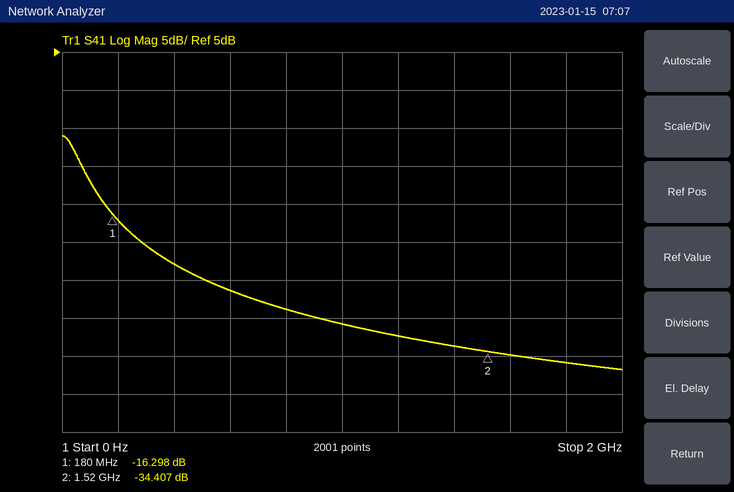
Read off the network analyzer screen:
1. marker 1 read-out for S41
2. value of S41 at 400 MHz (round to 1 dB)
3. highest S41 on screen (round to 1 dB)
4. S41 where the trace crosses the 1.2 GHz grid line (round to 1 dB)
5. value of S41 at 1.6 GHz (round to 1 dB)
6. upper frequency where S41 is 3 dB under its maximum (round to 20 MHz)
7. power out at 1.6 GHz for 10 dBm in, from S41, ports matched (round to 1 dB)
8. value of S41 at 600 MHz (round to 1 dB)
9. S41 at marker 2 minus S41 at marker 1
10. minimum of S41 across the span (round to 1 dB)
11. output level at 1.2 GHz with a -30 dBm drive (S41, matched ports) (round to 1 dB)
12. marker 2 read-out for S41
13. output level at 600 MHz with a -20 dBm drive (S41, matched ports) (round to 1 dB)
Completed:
-16.298 dB
-23 dB
-6 dB
-32 dB
-35 dB
60 MHz
-25 dBm
-26 dB
-18.109 dB
-37 dB
-62 dBm
-34.407 dB
-46 dBm
